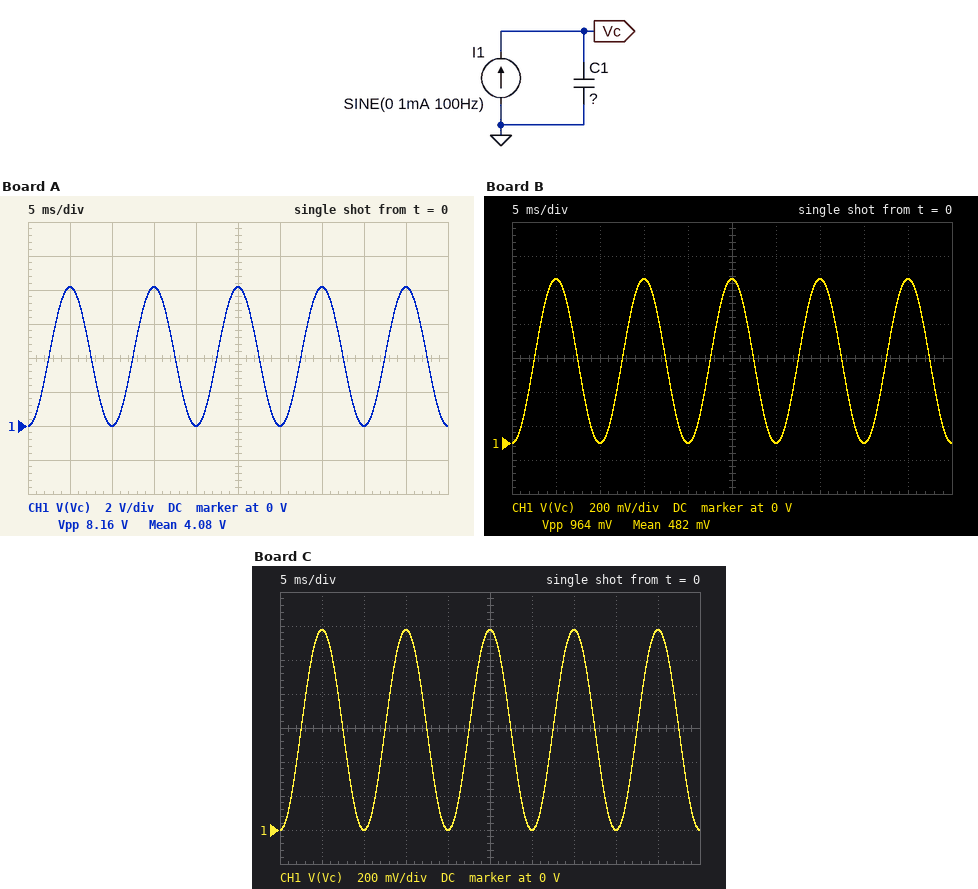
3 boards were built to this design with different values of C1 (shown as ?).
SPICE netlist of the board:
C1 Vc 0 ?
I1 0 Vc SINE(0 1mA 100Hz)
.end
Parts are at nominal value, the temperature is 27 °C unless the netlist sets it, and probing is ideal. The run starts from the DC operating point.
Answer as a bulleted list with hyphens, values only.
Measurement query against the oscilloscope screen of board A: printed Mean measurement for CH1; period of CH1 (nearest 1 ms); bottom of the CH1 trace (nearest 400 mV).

- 4.08 V
- 10 ms
- 0 V
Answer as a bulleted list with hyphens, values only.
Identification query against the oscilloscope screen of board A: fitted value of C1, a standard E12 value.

- 390 nF
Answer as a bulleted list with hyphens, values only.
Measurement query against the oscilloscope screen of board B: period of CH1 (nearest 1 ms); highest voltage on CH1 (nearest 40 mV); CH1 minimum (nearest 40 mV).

- 10 ms
- 960 mV
- 0 V
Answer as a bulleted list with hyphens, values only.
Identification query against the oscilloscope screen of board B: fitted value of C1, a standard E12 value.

- 3.3 µF
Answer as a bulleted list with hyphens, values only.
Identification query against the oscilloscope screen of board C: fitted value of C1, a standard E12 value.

- 2.7 µF
